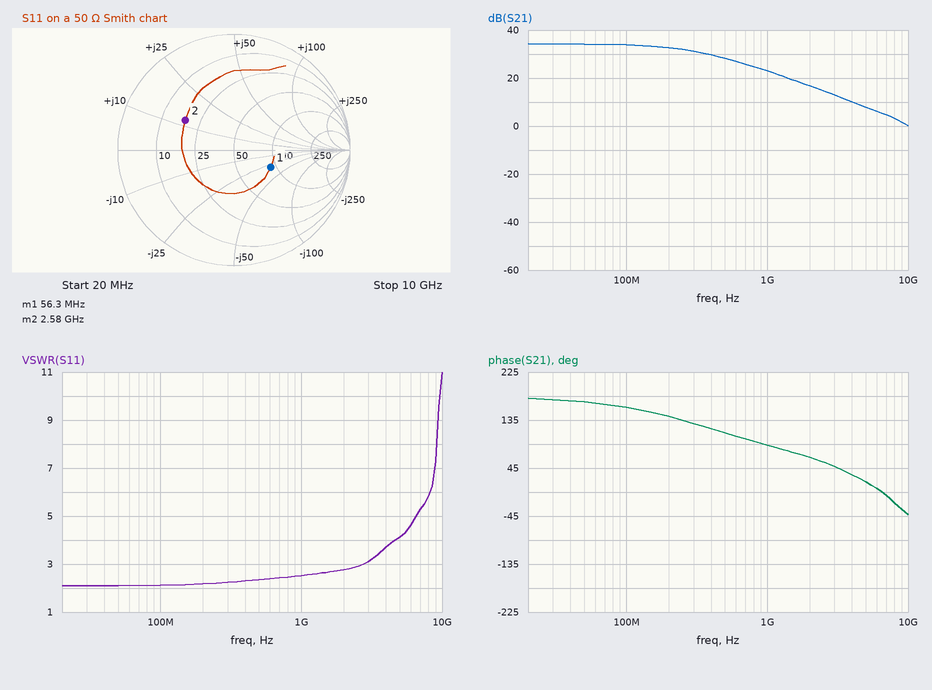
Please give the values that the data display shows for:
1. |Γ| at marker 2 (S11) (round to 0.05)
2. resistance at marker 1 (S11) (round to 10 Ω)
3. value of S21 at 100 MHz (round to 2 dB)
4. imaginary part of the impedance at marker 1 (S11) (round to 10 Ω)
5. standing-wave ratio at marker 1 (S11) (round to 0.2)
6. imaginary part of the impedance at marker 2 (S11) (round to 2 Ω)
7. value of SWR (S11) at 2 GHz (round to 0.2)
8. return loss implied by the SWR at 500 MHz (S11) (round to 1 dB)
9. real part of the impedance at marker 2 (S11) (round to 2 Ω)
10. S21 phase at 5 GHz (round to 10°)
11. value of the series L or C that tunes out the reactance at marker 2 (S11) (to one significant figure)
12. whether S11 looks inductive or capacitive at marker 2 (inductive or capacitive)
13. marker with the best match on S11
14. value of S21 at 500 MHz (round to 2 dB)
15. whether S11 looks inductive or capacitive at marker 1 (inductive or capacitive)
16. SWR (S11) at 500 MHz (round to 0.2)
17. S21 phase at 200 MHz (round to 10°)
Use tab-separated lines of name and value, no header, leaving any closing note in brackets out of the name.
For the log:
|Γ| at marker 2 (S11)	0.50
resistance at marker 1 (S11)	90 Ω
value of S21 at 100 MHz	34 dB
imaginary part of the impedance at marker 1 (S11)	-30 Ω
standing-wave ratio at marker 1 (S11)	2.0
imaginary part of the impedance at marker 2 (S11)	+12 Ω
value of SWR (S11) at 2 GHz	2.8
return loss implied by the SWR at 500 MHz (S11)	8 dB
real part of the impedance at marker 2 (S11)	18 Ω
S21 phase at 5 GHz	20°
value of the series L or C that tunes out the reactance at marker 2 (S11)	5 pF
whether S11 looks inductive or capacitive at marker 2	inductive
marker with the best match on S11	marker 1
value of S21 at 500 MHz	28 dB
whether S11 looks inductive or capacitive at marker 1	capacitive
SWR (S11) at 500 MHz	2.4
S21 phase at 200 MHz	140°
